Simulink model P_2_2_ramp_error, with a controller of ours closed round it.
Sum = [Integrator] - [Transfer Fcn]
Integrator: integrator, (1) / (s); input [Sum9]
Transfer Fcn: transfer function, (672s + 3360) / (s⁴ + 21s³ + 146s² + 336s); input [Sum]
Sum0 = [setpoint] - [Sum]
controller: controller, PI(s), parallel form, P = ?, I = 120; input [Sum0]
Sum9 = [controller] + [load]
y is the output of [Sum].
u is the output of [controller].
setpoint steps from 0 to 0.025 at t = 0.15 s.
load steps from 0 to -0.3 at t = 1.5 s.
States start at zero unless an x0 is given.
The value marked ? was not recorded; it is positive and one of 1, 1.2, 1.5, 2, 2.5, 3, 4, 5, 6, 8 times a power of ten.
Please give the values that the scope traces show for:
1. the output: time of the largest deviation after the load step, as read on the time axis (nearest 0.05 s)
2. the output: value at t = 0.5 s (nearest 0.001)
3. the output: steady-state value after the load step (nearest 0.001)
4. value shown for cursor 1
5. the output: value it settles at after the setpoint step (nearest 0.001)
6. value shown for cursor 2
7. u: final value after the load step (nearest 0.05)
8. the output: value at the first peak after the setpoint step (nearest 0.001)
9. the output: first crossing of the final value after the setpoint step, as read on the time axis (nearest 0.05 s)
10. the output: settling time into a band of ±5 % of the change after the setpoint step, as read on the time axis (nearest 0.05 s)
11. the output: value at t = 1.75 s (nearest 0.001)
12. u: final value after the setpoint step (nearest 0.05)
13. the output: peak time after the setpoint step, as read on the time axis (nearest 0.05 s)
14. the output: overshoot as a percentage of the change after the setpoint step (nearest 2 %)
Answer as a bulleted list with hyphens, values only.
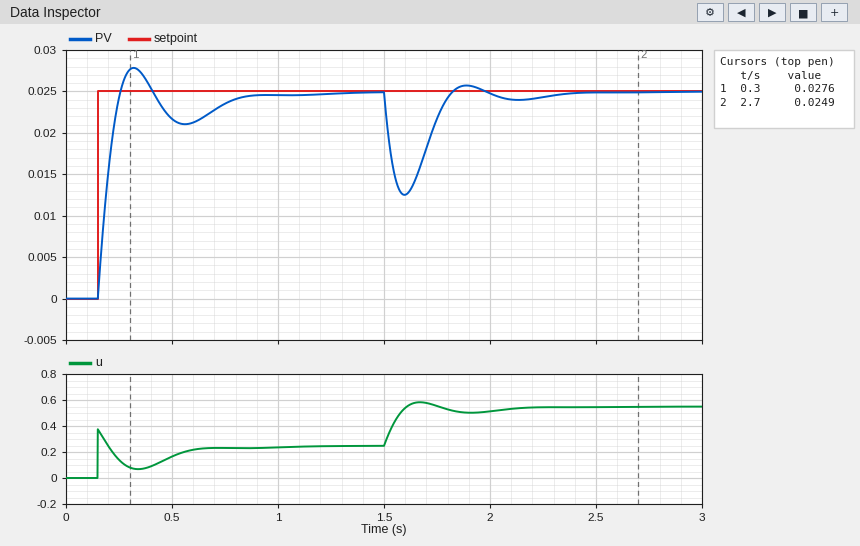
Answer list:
- 1.60 s
- 0.022
- 0.025
- 0.0276
- 0.025
- 0.0249
- 0.55
- 0.028
- 0.25 s
- 0.75 s
- 0.022
- 0.25
- 0.30 s
- 12 %
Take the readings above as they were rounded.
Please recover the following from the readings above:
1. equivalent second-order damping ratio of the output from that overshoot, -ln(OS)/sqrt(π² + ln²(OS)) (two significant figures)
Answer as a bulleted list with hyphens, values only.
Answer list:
- 0.56
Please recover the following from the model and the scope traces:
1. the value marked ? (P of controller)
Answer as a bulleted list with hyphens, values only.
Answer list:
- 15
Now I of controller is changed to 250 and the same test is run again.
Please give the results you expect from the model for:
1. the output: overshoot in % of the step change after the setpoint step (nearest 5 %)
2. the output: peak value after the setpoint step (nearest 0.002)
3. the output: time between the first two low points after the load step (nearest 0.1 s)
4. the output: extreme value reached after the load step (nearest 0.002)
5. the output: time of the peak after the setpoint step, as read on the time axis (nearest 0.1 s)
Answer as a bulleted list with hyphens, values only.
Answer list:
- 25 %
- 0.032
- 0.4 s
- 0.014
- 0.3 s
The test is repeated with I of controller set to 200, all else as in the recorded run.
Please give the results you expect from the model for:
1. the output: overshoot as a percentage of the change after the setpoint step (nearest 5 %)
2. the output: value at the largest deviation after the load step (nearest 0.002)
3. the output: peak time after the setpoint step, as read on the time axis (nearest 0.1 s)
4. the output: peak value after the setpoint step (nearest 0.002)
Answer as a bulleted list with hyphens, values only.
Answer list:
- 20 %
- 0.014
- 0.3 s
- 0.030
